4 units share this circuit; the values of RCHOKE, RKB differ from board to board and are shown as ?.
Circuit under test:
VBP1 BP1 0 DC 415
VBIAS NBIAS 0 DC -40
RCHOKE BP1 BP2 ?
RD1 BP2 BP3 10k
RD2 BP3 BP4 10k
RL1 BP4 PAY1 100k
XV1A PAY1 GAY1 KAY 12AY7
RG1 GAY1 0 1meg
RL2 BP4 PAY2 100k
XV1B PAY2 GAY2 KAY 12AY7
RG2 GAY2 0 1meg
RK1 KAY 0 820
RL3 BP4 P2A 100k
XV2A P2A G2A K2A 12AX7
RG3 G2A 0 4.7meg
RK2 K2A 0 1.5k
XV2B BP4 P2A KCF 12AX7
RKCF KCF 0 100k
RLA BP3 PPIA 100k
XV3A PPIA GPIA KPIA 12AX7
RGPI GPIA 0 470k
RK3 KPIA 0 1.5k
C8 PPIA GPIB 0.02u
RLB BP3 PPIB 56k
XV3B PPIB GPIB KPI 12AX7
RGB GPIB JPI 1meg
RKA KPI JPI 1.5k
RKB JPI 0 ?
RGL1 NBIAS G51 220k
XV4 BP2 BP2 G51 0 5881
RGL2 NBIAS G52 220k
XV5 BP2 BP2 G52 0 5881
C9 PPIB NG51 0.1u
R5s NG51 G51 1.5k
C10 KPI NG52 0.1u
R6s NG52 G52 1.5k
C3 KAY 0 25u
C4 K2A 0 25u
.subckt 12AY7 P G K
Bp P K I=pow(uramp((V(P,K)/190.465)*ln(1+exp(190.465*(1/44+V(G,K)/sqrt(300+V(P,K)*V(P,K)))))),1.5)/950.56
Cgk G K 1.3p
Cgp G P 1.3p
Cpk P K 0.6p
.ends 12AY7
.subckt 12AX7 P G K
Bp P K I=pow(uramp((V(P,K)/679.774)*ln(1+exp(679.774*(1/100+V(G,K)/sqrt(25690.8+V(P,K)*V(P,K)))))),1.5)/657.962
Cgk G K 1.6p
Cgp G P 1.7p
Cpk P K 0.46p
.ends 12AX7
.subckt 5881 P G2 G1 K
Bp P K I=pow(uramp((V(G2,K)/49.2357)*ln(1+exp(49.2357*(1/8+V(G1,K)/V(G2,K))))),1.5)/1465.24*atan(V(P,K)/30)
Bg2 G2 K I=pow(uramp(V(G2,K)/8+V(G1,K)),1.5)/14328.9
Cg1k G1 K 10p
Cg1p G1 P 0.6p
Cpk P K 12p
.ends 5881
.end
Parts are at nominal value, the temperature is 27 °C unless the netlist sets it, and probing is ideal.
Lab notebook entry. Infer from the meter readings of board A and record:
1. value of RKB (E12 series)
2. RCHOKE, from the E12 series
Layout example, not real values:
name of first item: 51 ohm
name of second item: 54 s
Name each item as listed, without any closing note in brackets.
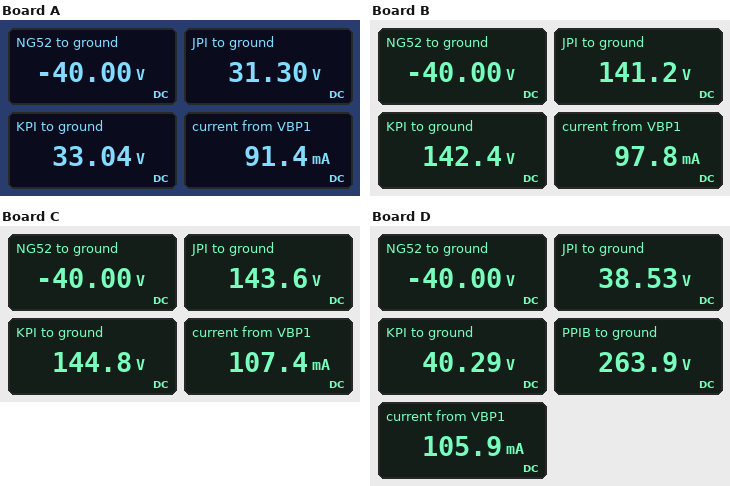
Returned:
value of RKB: 27 kΩ
RCHOKE, from the E12 series: 220 Ω
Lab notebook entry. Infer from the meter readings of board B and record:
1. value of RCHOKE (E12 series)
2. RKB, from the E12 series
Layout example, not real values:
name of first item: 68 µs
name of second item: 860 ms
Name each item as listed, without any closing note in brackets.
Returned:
value of RCHOKE: 150 Ω
RKB, from the E12 series: 180 kΩ
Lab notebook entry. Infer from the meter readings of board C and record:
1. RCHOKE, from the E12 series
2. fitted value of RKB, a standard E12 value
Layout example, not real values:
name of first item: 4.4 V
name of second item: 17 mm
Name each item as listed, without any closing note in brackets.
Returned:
RCHOKE, from the E12 series: 68 Ω
fitted value of RKB, a standard E12 value: 180 kΩ
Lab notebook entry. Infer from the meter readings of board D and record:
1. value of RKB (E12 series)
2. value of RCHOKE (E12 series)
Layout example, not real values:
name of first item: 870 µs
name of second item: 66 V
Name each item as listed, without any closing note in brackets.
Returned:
value of RKB: 33 kΩ
value of RCHOKE: 82 Ω
